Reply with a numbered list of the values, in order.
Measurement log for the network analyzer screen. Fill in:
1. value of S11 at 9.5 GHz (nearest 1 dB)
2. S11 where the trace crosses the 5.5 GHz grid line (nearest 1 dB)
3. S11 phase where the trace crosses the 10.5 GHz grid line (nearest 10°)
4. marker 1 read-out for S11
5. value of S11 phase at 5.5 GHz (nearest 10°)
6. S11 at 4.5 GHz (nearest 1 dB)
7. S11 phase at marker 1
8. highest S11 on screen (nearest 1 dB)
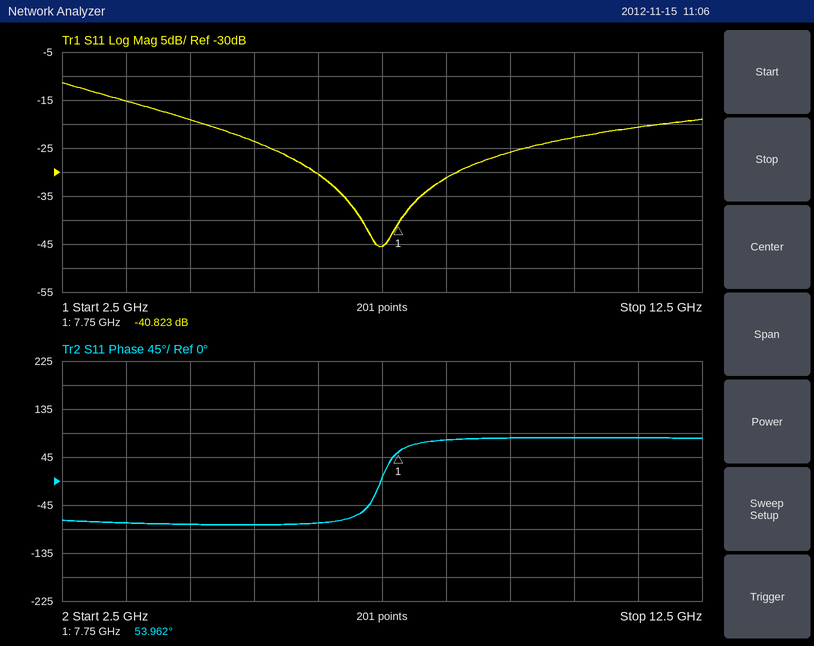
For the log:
1. -26 dB
2. -24 dB
3. 80°
4. -40.823 dB
5. -80°
6. -19 dB
7. 53.962°
8. -11 dB
